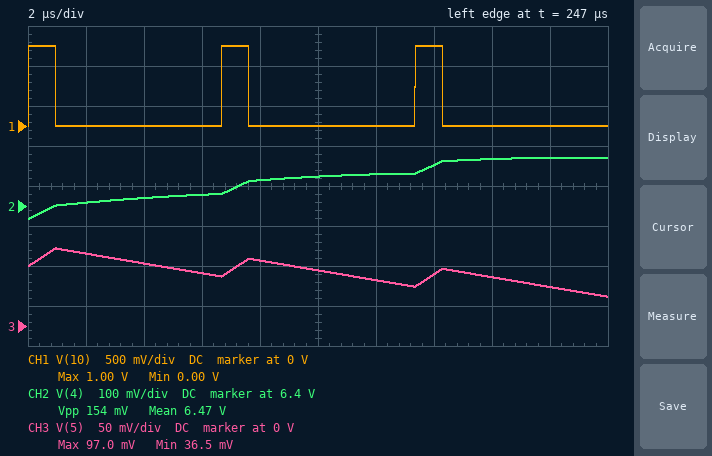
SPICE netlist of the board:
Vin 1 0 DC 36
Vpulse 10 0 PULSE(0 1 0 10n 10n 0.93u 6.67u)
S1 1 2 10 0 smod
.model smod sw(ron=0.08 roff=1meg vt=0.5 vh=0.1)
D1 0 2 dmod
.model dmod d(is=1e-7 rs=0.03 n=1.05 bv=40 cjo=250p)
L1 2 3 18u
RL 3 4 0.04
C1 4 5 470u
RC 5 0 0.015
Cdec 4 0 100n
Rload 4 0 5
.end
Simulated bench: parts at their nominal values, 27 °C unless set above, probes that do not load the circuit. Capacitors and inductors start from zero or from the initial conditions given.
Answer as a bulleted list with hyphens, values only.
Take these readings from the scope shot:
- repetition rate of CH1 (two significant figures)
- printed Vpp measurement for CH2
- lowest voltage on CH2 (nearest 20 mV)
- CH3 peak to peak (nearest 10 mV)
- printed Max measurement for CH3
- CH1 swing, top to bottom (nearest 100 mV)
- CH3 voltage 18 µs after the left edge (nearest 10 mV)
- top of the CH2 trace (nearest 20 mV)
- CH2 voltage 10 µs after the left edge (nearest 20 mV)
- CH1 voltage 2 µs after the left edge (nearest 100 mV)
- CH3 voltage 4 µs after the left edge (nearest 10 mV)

- 150 kHz
- 154 mV
- 6.36 V
- 60 mV
- 97.0 mV
- 1.0 V
- 50 mV
- 6.52 V
- 6.48 V
- 0 V
- 80 mV
